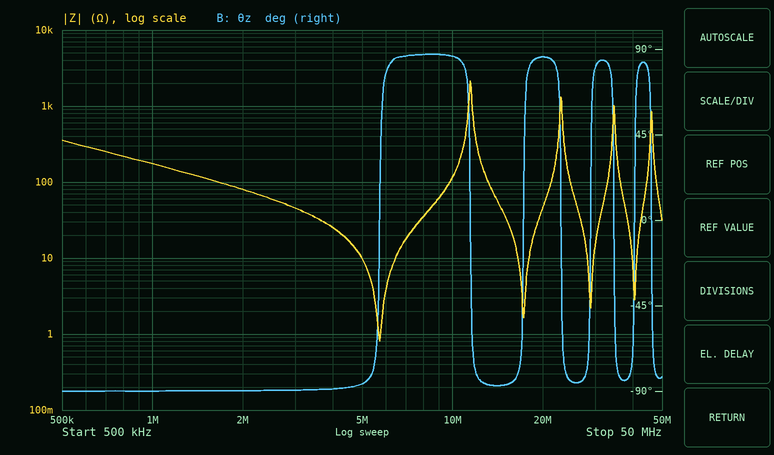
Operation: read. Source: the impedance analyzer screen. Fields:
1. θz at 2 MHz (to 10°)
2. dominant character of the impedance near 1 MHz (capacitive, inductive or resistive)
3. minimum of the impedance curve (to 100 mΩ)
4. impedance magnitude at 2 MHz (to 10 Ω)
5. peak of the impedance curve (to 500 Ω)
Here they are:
-90°
capacitive
800 mΩ
80 Ω
2.0 kΩ
